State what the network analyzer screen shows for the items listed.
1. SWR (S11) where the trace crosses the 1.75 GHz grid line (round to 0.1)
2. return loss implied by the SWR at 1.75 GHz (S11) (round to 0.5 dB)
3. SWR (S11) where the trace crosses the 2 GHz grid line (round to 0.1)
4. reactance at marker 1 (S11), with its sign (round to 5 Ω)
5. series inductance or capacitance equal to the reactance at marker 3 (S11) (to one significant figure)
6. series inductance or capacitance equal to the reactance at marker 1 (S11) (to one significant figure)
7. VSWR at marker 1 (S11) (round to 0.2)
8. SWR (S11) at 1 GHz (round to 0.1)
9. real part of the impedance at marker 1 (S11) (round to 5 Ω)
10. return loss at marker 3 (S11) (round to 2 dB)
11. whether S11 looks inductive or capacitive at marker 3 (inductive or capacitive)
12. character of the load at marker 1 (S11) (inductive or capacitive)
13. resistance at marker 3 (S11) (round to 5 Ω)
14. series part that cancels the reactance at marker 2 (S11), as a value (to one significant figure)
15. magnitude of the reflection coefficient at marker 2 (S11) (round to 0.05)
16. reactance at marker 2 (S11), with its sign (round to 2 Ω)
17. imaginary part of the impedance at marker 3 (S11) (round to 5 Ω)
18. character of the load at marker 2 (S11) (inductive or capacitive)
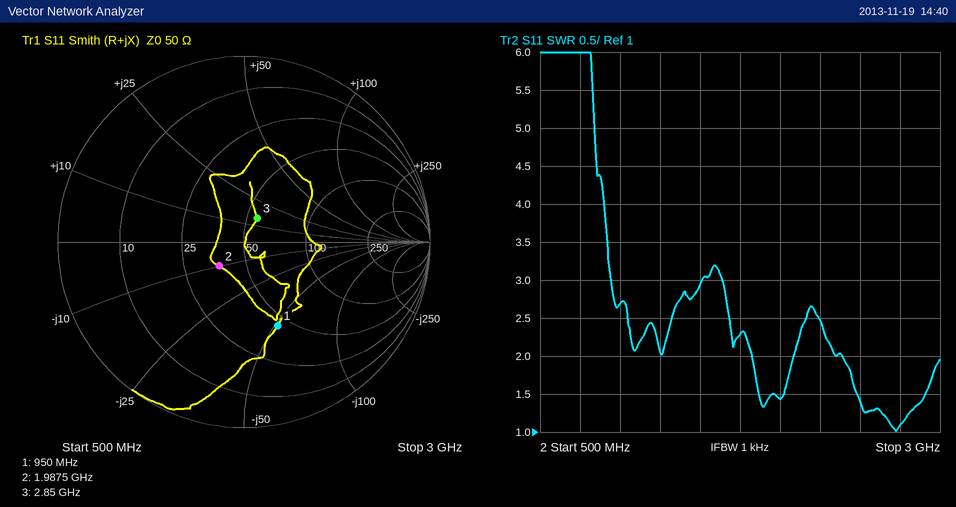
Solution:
2.3
8.0 dB
1.4
-50 Ω
800 pH
3 pF
2.8
2.7
45 Ω
16 dB
inductive
capacitive
55 Ω
800 pH
0.20
-10 Ω
+15 Ω
capacitive
